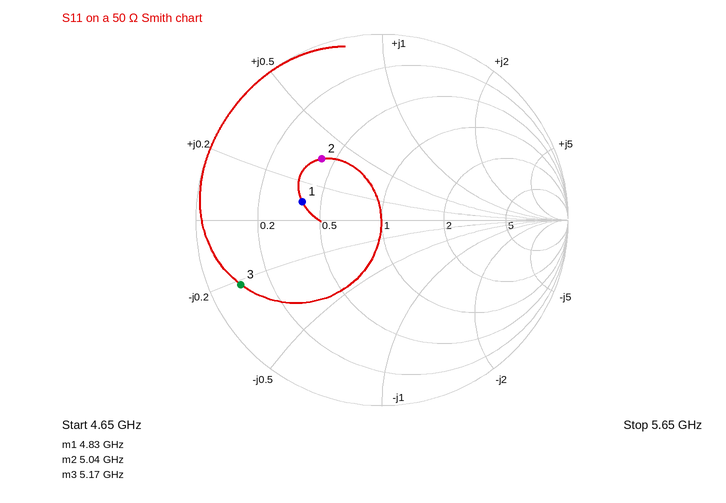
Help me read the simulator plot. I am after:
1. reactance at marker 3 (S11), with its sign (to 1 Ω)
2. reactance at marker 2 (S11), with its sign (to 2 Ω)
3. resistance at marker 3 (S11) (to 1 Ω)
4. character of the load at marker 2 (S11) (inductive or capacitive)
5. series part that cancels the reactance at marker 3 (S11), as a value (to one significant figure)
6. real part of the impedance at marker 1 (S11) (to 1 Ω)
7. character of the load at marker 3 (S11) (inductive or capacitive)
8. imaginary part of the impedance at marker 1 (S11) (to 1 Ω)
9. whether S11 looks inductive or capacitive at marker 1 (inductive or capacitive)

-11 Ω
+18 Ω
5 Ω
inductive
300 pH
20 Ω
capacitive
+5 Ω
inductive
